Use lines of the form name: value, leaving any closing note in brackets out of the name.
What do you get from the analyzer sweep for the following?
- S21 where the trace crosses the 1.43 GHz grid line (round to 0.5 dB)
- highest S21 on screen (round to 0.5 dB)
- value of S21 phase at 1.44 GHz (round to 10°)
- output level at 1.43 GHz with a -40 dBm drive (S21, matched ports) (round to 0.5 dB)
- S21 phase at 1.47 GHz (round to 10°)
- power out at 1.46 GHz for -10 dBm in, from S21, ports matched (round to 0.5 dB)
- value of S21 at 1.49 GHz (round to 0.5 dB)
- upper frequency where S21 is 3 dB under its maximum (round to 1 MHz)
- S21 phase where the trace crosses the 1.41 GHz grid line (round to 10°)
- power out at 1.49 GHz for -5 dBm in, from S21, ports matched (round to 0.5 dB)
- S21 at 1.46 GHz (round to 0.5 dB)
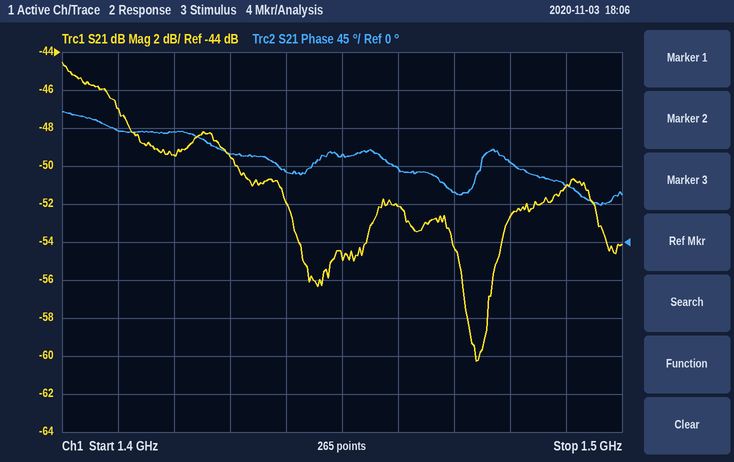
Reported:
S21 where the trace crosses the 1.43 GHz grid line: -49.5 dB
highest S21 on screen: -44.5 dB
value of S21 phase at 1.44 GHz: 80°
output level at 1.43 GHz with a -40 dBm drive (S21, matched ports): -89.5 dBm
S21 phase at 1.47 GHz: 60°
power out at 1.46 GHz for -10 dBm in, from S21, ports matched: -62.0 dBm
value of S21 at 1.49 GHz: -51.0 dB
upper frequency where S21 is 3 dB under its maximum: 1.411 GHz
S21 phase where the trace crosses the 1.41 GHz grid line: 130°
power out at 1.49 GHz for -5 dBm in, from S21, ports matched: -56.0 dBm
S21 at 1.46 GHz: -52.0 dB
